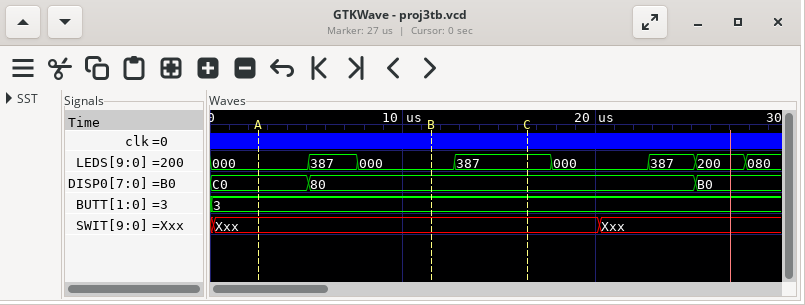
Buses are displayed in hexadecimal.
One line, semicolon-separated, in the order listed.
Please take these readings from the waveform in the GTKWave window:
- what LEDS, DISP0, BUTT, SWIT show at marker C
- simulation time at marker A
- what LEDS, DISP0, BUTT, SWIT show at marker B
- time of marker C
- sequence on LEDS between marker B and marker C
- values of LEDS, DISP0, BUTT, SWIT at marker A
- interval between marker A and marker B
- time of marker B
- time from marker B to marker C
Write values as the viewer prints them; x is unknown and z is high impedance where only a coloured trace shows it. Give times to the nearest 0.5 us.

LEDS=387, DISP0=80, BUTT=3, SWIT=Xxx; 2.5 us; LEDS=000, DISP0=80, BUTT=3, SWIT=Xxx; 16.5 us; 000, 387; LEDS=000, DISP0=C0, BUTT=3, SWIT=Xxx; 9 us; 11.5 us; 5 us
